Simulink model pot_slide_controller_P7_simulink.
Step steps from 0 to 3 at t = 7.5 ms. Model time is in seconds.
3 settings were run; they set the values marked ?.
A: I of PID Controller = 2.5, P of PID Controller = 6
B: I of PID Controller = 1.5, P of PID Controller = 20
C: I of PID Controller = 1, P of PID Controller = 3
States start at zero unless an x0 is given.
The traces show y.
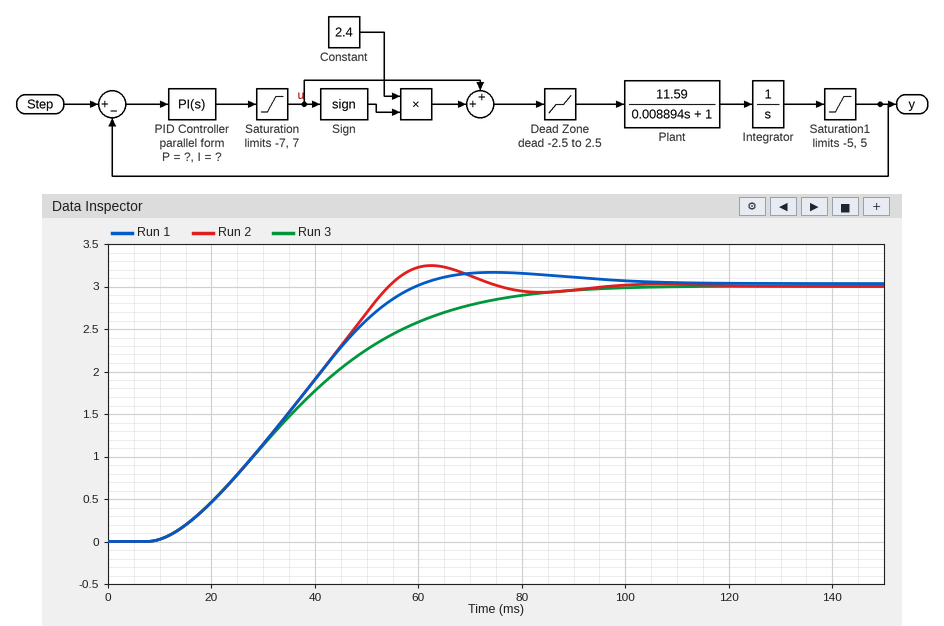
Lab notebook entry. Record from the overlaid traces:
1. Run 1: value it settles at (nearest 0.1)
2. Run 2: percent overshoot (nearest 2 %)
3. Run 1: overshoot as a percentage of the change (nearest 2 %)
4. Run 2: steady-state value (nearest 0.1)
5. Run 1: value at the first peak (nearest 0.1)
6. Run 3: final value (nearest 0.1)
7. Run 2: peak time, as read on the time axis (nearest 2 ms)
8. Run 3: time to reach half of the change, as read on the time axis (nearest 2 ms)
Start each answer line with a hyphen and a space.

- 3.0
- 8 %
- 4 %
- 3.0
- 3.2
- 3.0
- 62 ms
- 36 ms
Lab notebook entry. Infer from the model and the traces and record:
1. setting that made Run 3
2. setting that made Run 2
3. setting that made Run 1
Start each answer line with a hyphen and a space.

- C
- B
- A
